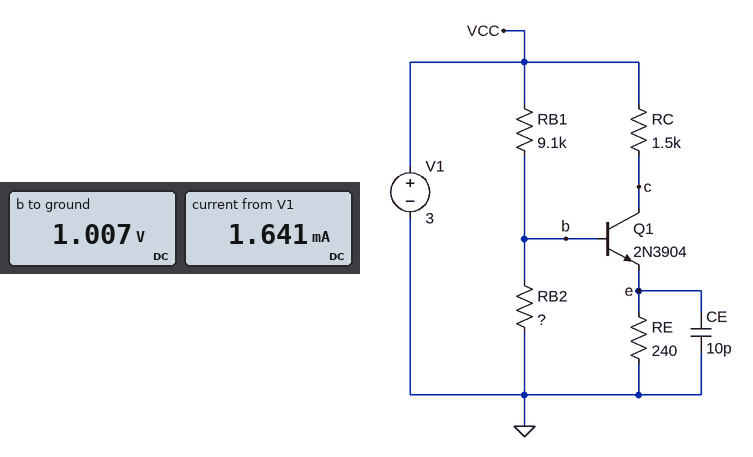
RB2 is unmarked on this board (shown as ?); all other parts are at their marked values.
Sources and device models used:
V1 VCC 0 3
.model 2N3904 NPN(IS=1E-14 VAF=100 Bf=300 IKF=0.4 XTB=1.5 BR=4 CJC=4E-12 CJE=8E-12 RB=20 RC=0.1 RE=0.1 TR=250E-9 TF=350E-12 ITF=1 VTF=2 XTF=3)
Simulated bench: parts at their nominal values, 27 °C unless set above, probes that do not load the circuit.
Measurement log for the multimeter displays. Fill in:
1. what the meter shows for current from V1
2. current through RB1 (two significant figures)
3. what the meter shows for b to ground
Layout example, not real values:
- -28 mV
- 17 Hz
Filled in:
- 1.641 mA
- 220 µA
- 1.007 V
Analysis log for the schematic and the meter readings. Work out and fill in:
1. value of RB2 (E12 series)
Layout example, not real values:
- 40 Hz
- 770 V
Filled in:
- 4.7 kΩ
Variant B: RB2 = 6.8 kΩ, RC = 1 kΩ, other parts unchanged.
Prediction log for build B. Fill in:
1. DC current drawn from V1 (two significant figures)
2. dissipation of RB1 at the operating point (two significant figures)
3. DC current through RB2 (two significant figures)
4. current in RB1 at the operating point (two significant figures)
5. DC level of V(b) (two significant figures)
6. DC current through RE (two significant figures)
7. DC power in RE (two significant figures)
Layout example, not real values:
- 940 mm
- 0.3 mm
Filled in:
- 2.5 mA
- 340 µW
- 180 µA
- 190 µA
- 1.2 V
- 2.3 mA
- 1.3 mW
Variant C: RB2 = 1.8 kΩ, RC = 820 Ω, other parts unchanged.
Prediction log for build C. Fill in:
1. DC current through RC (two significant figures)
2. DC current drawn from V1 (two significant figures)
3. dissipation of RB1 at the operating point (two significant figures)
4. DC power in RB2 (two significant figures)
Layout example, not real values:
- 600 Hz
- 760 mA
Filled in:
- 2.1 µA
- 280 µA
- 690 µW
- 140 µW
